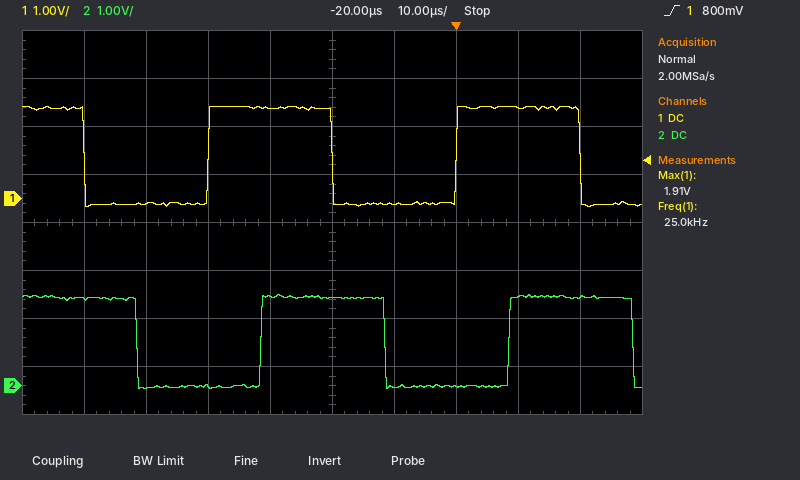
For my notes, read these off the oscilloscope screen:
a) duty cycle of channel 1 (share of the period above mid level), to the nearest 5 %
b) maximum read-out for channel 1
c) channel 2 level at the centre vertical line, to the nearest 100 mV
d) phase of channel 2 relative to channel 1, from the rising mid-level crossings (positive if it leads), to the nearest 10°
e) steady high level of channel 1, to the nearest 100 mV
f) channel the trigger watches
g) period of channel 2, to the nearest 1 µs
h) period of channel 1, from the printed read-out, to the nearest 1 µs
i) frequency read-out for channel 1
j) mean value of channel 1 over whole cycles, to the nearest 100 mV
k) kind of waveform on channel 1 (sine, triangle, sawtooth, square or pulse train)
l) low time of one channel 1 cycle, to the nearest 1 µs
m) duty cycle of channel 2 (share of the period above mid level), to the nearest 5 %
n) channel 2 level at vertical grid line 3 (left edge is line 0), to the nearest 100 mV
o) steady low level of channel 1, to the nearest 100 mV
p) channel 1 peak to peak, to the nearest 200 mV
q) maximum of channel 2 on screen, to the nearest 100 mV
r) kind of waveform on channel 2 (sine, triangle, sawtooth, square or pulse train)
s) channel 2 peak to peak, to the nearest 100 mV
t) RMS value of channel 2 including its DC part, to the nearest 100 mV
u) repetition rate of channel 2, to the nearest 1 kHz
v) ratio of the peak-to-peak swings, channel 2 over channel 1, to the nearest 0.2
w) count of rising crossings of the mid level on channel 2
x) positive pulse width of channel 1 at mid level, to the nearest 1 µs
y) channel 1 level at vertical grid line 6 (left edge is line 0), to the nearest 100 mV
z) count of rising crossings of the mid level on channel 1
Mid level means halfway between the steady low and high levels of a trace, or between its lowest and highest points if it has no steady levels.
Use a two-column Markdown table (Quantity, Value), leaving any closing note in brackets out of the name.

| Quantity | Value |
|---|---|
| duty cycle of channel 1 (share of the period above mid level), to the nearest 5 % | 50 % |
| maximum read-out for channel 1 | 1.91 V |
| channel 2 level at the centre vertical line, to the nearest 100 mV | 1.8 V |
| phase of channel 2 relative to channel 1, from the rising mid-level crossings (positive if it leads), to the nearest 10° | -80° |
| steady high level of channel 1, to the nearest 100 mV | 1.9 V |
| channel the trigger watches | channel 1 |
| period of channel 2, to the nearest 1 µs | 40 µs |
| period of channel 1, from the printed read-out, to the nearest 1 µs | 40 µs |
| frequency read-out for channel 1 | 25.0 kHz |
| mean value of channel 1 over whole cycles, to the nearest 100 mV | 900 mV |
| kind of waveform on channel 1 | square |
| low time of one channel 1 cycle, to the nearest 1 µs | 20 µs |
| duty cycle of channel 2 (share of the period above mid level), to the nearest 5 % | 50 % |
| channel 2 level at vertical grid line 3 (left edge is line 0), to the nearest 100 mV | 0.0 V |
| steady low level of channel 1, to the nearest 100 mV | -100 mV |
| channel 1 peak to peak, to the nearest 200 mV | 2.0 V |
| maximum of channel 2 on screen, to the nearest 100 mV | 1.9 V |
| kind of waveform on channel 2 | square |
| channel 2 peak to peak, to the nearest 100 mV | 2.0 V |
| RMS value of channel 2 including its DC part, to the nearest 100 mV | 1.3 V |
| repetition rate of channel 2, to the nearest 1 kHz | 25 kHz |
| ratio of the peak-to-peak swings, channel 2 over channel 1, to the nearest 0.2 | 1.0 |
| count of rising crossings of the mid level on channel 2 | 2 |
| positive pulse width of channel 1 at mid level, to the nearest 1 µs | 20 µs |
| channel 1 level at vertical grid line 6 (left edge is line 0), to the nearest 100 mV | -100 mV |
| count of rising crossings of the mid level on channel 1 | 2 |
